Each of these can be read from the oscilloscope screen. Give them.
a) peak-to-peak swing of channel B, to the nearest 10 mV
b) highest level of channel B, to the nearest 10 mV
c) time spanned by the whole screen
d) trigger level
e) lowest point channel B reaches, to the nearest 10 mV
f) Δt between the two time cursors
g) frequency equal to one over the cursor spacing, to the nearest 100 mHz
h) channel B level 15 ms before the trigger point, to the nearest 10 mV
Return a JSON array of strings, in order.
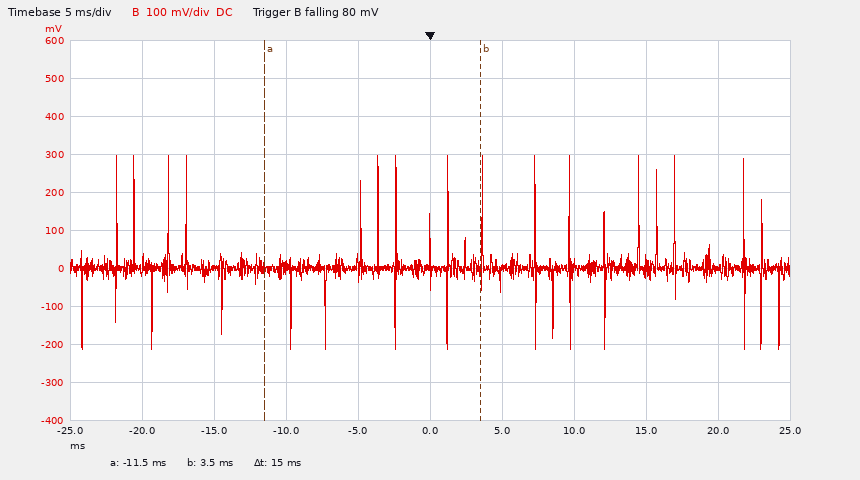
["510 mV", "300 mV", "50 ms", "80 mV", "-210 mV", "15 ms", "66.7 Hz", "0 mV"]
